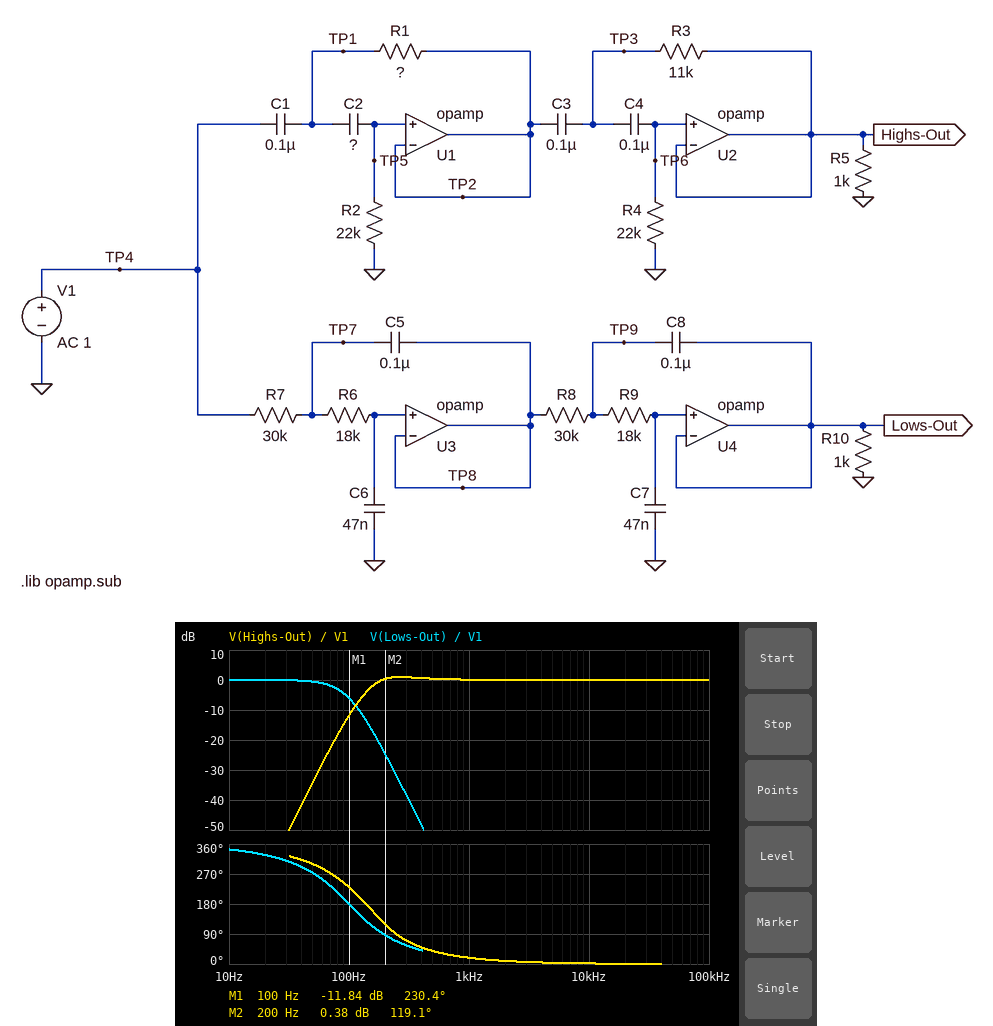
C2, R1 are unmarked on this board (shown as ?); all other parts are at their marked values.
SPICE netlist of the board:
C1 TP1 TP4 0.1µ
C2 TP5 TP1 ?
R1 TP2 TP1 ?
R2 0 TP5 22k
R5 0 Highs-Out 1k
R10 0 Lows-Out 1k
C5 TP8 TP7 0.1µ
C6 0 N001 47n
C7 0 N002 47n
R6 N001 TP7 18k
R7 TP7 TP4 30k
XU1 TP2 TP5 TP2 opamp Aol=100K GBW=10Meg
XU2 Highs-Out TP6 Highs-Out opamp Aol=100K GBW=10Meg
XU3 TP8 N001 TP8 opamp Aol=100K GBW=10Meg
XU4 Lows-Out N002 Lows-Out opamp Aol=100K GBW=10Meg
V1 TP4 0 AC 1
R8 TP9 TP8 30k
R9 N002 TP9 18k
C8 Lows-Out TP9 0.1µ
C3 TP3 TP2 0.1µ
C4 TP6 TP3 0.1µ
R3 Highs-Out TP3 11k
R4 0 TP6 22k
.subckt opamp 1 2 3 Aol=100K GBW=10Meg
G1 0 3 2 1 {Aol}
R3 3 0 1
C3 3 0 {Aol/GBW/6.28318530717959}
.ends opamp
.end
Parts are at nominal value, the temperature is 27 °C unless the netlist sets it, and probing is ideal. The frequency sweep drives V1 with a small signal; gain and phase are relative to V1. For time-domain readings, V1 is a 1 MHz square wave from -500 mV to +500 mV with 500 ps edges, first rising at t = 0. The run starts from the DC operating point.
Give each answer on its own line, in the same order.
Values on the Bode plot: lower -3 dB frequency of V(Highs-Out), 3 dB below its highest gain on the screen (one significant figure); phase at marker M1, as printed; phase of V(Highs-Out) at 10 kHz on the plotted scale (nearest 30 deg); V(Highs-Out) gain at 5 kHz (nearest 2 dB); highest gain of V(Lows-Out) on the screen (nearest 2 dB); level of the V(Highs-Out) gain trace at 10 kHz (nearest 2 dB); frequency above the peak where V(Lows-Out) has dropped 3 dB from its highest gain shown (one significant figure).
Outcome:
200 Hz
230.4 deg
0 deg
0 dB
0 dB
0 dB
80 Hz
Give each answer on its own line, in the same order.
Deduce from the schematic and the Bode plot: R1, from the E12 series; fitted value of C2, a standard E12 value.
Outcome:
5.6 kΩ
68 nF
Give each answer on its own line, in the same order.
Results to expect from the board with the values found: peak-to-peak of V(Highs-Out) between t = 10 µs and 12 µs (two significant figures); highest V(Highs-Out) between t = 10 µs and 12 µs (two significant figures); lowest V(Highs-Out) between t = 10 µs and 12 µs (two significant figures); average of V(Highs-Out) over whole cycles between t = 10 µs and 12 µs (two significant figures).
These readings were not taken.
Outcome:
1.0 V
990 mV
-12 mV
490 mV
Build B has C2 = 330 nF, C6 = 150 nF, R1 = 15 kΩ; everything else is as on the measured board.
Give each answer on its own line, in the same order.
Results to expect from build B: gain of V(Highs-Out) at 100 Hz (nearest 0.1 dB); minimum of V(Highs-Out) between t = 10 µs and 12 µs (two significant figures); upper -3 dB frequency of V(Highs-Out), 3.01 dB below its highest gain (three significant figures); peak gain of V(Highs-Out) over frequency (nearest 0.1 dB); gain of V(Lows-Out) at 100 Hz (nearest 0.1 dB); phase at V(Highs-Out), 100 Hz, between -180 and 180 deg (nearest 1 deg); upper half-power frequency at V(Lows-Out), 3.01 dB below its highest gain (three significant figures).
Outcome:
-4.9 dB
-9.0 mV
6.44 MHz
0 dB
-17.1 dB
143 deg
25.9 Hz
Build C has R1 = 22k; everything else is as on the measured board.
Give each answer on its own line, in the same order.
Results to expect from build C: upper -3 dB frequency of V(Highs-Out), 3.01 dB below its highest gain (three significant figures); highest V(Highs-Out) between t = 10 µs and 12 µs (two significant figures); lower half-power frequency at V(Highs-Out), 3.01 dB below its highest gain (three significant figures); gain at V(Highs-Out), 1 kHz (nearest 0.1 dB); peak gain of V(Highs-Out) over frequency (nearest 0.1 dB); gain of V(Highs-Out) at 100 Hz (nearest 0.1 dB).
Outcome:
6.44 MHz
990 mV
161 Hz
-0.1 dB
0 dB
-8.3 dB
